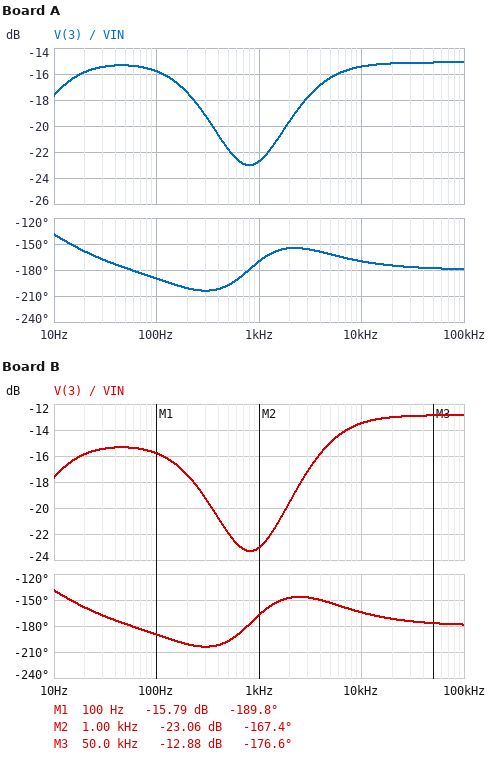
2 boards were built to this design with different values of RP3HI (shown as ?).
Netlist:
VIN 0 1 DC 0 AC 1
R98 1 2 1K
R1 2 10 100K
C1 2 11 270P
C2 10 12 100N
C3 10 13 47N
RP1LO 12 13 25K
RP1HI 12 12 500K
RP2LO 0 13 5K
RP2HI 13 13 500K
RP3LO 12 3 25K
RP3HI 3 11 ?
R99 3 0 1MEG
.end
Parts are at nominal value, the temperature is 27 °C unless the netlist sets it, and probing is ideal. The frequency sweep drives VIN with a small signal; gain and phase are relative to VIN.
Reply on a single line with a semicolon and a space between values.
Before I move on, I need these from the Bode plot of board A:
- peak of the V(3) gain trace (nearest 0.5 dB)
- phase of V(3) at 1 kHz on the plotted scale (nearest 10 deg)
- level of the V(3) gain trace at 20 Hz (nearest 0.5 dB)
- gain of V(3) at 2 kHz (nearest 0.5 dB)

-15.0 dB; -170 deg; -16.0 dB; -19.5 dB
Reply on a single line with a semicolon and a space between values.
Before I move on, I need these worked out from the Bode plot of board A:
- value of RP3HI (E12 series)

180 kΩ
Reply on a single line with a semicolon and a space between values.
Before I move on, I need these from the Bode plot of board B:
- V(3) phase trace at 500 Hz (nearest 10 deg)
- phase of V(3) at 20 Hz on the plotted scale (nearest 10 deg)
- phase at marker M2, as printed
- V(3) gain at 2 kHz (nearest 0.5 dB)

-200 deg; -160 deg; -167.4 deg; -19.5 dB
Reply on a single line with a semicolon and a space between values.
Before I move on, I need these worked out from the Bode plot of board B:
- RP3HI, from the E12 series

120 kΩ
